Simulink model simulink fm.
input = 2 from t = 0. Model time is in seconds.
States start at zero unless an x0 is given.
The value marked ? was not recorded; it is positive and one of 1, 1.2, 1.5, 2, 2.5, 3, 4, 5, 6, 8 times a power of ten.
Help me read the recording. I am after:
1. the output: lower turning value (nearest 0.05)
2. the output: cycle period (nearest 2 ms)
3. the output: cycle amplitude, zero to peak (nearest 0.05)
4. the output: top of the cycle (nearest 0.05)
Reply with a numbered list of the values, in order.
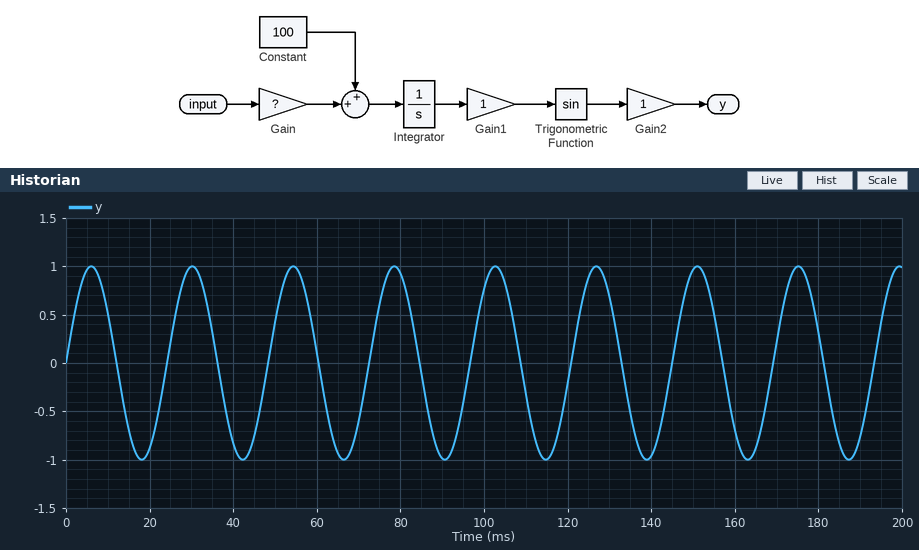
1. -1.00
2. 24 ms
3. 1.00
4. 1.00
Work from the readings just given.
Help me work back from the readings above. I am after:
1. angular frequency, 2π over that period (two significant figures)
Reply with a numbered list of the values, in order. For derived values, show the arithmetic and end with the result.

1. 2π / 24 = 0.26 rad/ms
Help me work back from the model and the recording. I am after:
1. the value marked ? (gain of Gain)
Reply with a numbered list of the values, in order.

1. 80
